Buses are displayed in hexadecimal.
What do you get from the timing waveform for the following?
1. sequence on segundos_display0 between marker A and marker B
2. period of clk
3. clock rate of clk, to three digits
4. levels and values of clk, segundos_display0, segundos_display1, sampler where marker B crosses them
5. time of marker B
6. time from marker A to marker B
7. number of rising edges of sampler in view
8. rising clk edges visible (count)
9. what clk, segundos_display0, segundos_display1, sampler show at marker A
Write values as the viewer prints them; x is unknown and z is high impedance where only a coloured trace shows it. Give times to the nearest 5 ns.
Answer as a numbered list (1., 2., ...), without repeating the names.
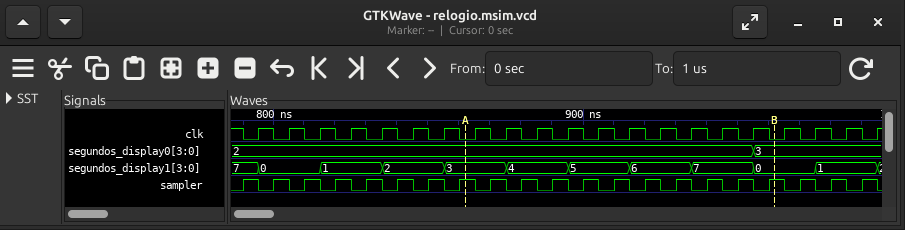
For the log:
1. 2, 3
2. 10 ns
3. 100 MHz
4. clk=0, segundos_display0=3, segundos_display1=0, sampler=1
5. 960 ns
6. 100 ns
7. 21
8. 21
9. clk=0, segundos_display0=2, segundos_display1=3, sampler=1
